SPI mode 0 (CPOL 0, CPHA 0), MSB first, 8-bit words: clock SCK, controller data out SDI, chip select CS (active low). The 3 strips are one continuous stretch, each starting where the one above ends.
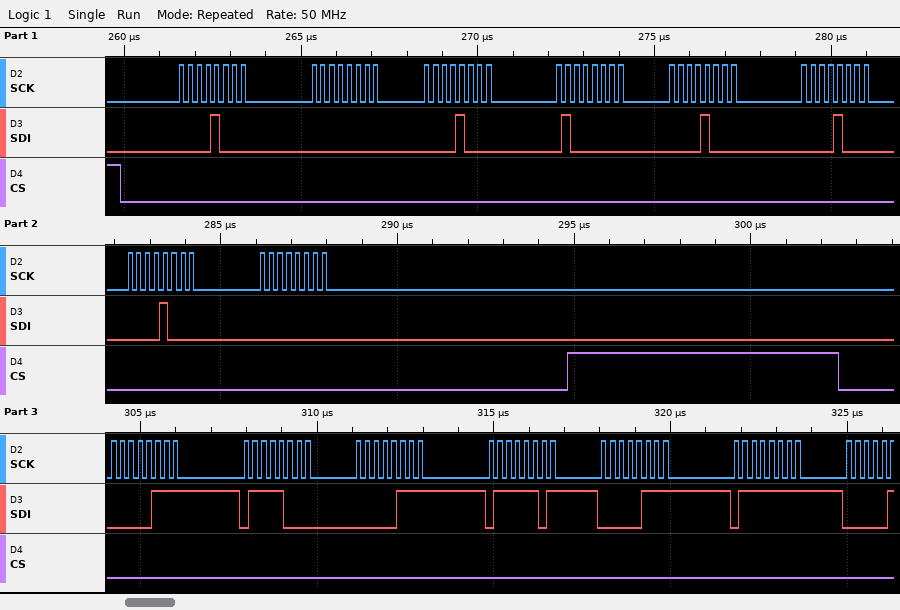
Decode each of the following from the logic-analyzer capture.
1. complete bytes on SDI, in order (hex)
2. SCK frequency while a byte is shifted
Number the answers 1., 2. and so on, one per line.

1. 0x08 0x00 0x08 0x40 0x08 0x08 0x08 0x00 0x07 0x78 0x07 0x7D 0x07 0x7F
2. 4 MHz
